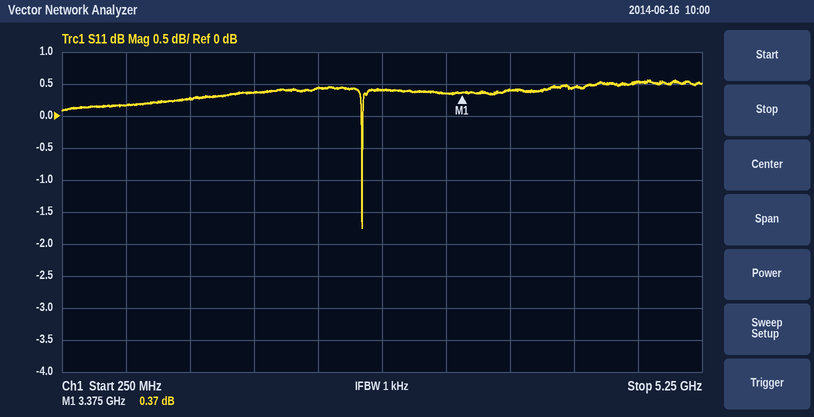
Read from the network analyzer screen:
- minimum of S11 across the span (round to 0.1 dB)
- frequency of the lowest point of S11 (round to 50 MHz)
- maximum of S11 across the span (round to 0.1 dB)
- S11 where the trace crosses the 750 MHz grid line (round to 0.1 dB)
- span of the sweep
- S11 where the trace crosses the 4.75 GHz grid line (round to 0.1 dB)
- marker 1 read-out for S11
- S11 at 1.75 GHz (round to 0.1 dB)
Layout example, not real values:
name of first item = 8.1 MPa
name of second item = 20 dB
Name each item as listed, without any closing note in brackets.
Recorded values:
minimum of S11 across the span = -1.8 dB
frequency of the lowest point of S11 = 2.60 GHz
maximum of S11 across the span = 0.6 dB
S11 where the trace crosses the 750 MHz grid line = 0.2 dB
span of the sweep = 5 GHz
S11 where the trace crosses the 4.75 GHz grid line = 0.5 dB
marker 1 read-out for S11 = 0.37 dB
S11 at 1.75 GHz = 0.4 dB
